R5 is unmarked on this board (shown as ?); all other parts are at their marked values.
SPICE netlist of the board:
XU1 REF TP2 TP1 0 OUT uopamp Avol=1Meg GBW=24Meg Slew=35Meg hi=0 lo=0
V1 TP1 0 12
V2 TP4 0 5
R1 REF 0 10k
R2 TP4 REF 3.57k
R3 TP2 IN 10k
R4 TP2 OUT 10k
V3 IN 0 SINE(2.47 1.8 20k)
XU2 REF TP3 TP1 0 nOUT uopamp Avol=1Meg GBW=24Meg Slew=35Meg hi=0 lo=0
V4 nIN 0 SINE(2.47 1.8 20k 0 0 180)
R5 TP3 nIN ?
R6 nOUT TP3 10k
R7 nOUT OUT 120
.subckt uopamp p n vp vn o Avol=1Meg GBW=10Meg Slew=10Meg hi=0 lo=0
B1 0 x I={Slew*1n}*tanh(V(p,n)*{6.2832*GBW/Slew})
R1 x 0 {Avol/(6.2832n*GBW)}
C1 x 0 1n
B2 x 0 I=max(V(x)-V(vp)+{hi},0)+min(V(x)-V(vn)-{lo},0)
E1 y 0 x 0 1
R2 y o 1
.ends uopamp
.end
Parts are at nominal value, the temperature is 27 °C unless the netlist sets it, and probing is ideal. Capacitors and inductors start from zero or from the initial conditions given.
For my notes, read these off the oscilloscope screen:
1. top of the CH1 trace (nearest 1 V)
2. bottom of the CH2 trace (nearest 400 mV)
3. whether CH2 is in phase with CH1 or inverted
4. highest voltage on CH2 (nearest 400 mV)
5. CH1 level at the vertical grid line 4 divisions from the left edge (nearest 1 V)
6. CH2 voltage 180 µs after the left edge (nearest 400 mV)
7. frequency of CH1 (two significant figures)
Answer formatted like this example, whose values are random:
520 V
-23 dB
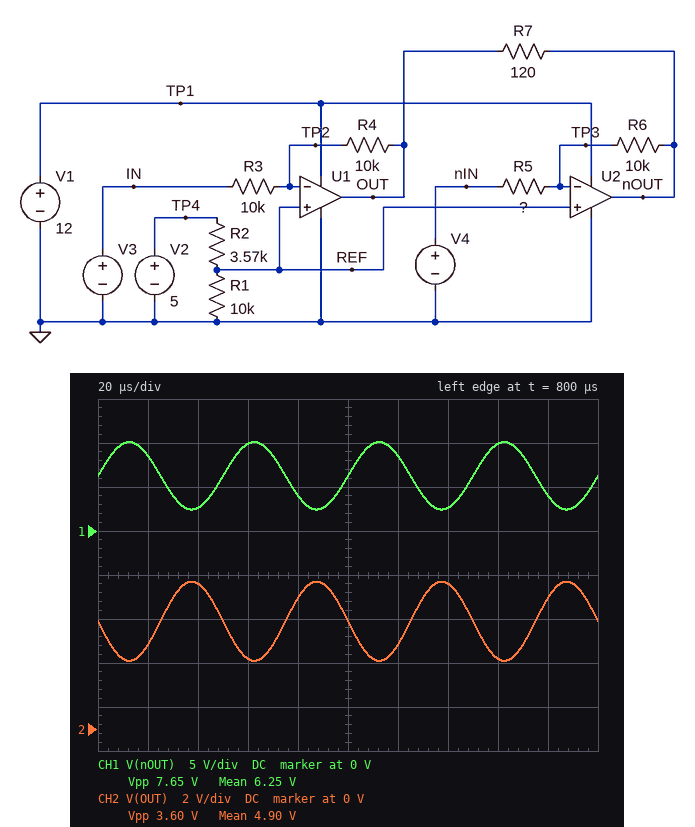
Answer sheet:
10 V
3.2 V
inverted
6.8 V
4 V
6.0 V
20 kHz
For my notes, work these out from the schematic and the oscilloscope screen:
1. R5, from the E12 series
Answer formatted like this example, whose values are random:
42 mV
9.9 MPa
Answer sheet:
4.7 kΩ
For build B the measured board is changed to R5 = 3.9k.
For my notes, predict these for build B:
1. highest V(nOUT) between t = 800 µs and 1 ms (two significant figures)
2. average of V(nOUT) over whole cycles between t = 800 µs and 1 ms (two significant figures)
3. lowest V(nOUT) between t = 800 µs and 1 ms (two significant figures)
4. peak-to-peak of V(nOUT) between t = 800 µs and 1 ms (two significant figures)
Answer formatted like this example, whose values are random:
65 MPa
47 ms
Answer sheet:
11 V
6.8 V
2.2 V
9.2 V
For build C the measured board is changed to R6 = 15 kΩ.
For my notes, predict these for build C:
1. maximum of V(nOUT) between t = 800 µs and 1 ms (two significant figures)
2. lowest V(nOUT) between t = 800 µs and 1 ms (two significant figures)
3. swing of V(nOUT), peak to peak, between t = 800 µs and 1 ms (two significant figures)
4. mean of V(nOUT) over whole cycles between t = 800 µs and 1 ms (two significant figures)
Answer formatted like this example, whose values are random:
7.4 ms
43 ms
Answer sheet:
12 V
1.8 V
10 V
7.4 V
